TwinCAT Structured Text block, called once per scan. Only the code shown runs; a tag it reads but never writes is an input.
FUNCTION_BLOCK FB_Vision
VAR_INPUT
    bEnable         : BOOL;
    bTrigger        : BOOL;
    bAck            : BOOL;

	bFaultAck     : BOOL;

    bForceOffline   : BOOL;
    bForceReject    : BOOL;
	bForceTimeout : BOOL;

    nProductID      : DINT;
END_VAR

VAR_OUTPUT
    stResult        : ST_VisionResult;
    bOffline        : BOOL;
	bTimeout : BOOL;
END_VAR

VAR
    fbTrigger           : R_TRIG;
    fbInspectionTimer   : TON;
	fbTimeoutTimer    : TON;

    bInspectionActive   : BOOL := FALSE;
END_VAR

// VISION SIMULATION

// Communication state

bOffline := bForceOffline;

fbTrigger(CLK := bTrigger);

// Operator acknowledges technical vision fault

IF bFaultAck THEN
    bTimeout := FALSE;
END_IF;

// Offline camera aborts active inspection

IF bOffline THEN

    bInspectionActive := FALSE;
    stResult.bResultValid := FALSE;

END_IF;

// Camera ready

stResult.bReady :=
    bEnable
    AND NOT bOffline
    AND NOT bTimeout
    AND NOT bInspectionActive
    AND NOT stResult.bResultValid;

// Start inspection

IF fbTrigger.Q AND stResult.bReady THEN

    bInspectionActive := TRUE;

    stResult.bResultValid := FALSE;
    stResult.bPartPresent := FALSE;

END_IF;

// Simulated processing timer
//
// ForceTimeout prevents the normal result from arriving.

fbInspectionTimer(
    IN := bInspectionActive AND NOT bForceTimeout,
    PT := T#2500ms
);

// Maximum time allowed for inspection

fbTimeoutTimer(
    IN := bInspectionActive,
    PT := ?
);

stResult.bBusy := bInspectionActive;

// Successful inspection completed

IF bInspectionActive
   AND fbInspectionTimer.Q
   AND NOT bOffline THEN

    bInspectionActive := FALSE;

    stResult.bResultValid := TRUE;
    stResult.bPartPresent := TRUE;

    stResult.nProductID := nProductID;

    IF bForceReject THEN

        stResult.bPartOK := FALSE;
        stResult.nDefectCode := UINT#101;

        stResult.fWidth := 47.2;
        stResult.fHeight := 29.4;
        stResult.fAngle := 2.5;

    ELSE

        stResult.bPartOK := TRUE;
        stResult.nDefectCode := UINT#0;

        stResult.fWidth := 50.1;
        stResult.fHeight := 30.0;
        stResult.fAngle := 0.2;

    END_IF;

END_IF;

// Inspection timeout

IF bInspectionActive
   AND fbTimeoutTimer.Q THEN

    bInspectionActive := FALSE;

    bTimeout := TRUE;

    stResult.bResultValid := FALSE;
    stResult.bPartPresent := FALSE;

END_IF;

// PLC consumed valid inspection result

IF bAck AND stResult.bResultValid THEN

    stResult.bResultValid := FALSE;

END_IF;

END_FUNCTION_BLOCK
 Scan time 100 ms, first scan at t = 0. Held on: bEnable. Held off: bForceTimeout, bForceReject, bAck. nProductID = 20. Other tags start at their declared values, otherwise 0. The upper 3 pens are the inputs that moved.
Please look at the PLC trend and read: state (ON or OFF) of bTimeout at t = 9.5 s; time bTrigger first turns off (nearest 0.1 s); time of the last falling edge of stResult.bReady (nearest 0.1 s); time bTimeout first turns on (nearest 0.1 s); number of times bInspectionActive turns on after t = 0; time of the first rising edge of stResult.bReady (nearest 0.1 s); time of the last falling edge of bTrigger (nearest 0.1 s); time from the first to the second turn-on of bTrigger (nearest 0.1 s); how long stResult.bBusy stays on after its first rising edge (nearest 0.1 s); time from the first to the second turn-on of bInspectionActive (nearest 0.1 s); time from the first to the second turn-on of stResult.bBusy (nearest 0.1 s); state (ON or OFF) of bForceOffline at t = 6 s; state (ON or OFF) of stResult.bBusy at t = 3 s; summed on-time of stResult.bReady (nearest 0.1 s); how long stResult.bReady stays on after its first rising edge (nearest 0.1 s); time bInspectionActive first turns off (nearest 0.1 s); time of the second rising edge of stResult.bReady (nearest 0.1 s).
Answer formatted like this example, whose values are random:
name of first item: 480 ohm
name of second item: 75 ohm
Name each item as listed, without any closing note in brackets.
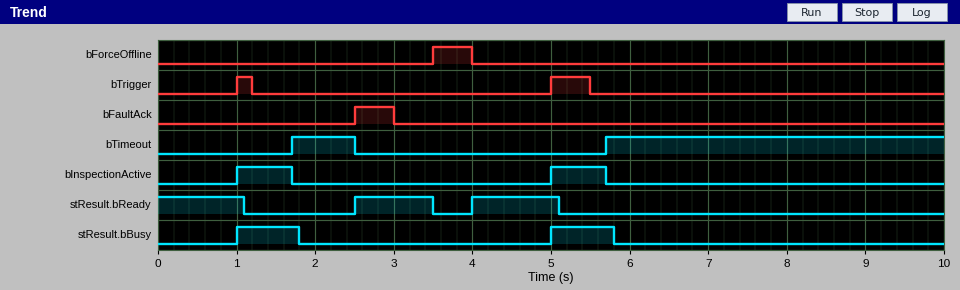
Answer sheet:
state (ON or OFF) of bTimeout at t = 9.5 s: ON
time bTrigger first turns off: 1.2 s
time of the last falling edge of stResult.bReady: 5.1 s
time bTimeout first turns on: 1.7 s
number of times bInspectionActive turns on after t = 0: 2
time of the first rising edge of stResult.bReady: 2.5 s
time of the last falling edge of bTrigger: 5.5 s
time from the first to the second turn-on of bTrigger: 4.0 s
how long stResult.bBusy stays on after its first rising edge: 0.8 s
time from the first to the second turn-on of bInspectionActive: 4.0 s
time from the first to the second turn-on of stResult.bBusy: 4.0 s
state (ON or OFF) of bForceOffline at t = 6 s: OFF
state (ON or OFF) of stResult.bBusy at t = 3 s: OFF
summed on-time of stResult.bReady: 3.2 s
how long stResult.bReady stays on after its first rising edge: 1.0 s
time bInspectionActive first turns off: 1.7 s
time of the second rising edge of stResult.bReady: 4.0 s
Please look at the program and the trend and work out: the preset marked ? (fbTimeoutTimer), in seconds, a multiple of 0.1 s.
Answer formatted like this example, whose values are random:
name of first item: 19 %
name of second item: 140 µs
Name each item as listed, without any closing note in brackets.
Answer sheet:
the preset marked ? (fbTimeoutTimer), in seconds, a multiple of 0.1 s: 0.7 s
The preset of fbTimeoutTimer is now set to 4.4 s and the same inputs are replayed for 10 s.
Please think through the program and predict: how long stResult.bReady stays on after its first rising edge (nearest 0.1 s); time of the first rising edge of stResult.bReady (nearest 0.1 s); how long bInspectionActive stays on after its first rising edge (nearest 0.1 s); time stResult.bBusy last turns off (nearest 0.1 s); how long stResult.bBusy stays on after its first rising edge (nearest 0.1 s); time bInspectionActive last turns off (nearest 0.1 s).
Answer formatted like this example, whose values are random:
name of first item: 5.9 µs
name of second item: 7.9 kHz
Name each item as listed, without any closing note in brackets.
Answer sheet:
how long stResult.bReady stays on after its first rising edge: 1.1 s
time of the first rising edge of stResult.bReady: 4.0 s
how long bInspectionActive stays on after its first rising edge: 2.5 s
time stResult.bBusy last turns off: 7.6 s
how long stResult.bBusy stays on after its first rising edge: 2.5 s
time bInspectionActive last turns off: 7.5 s
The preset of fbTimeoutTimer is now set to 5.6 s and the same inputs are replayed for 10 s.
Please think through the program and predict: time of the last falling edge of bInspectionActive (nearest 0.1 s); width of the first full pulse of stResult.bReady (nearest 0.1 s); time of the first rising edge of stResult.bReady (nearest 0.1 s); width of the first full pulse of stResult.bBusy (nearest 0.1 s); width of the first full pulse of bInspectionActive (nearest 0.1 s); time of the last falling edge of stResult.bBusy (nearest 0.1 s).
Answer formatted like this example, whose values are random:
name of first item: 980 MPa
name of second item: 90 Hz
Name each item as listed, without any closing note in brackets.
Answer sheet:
time of the last falling edge of bInspectionActive: 7.5 s
width of the first full pulse of stResult.bReady: 1.1 s
time of the first rising edge of stResult.bReady: 4.0 s
width of the first full pulse of stResult.bBusy: 2.5 s
width of the first full pulse of bInspectionActive: 2.5 s
time of the last falling edge of stResult.bBusy: 7.6 s
